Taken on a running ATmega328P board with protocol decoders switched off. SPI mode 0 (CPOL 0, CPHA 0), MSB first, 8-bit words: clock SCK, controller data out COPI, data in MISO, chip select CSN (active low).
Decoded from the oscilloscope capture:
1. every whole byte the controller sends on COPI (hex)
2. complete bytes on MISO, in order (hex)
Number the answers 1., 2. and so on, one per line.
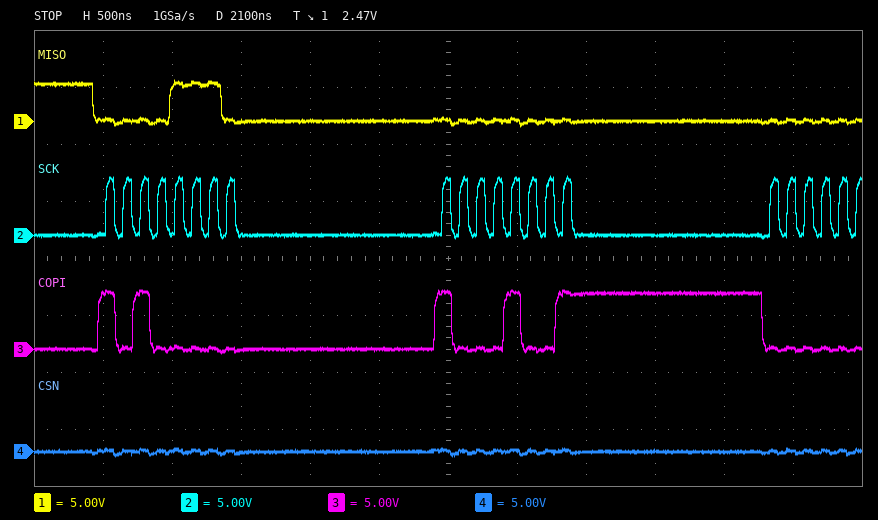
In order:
1. A0 89
2. 0E 00
